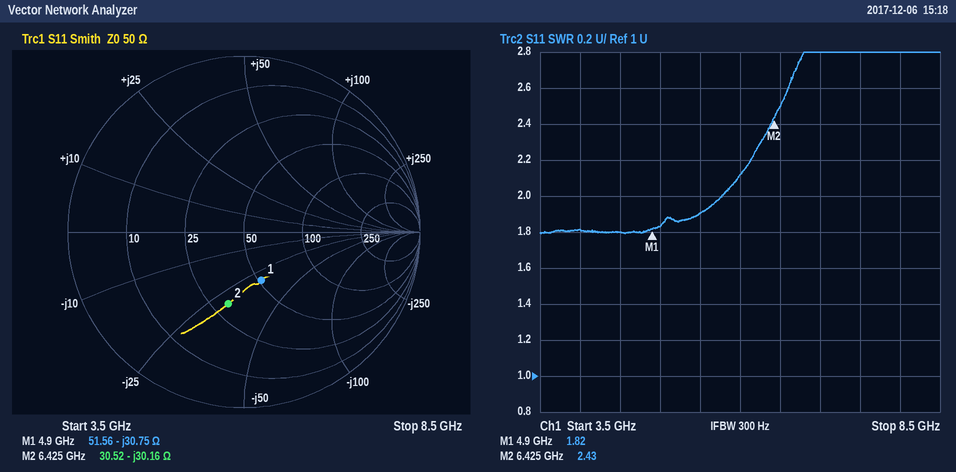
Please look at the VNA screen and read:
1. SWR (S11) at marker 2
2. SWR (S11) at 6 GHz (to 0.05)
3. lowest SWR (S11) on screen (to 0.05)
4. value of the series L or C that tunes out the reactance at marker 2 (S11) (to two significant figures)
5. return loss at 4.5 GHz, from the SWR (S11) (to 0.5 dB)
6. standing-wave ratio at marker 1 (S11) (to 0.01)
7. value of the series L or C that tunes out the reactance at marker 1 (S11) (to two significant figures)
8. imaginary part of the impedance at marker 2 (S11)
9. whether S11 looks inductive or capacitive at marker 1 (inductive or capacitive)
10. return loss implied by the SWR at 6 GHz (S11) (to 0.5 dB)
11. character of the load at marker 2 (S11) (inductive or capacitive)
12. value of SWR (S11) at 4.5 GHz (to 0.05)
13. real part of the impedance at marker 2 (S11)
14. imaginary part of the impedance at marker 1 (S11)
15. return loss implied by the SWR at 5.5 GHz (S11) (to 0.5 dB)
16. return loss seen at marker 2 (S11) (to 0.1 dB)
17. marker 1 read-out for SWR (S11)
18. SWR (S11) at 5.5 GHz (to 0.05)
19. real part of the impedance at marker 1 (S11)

2.43
2.10
1.80
750 pH
11.0 dB
1.82
1.00 nH
-30.16 Ω
capacitive
9.0 dB
capacitive
1.80
30.52 Ω
-30.75 Ω
10.0 dB
7.6 dB
1.82
1.90
51.56 Ω
